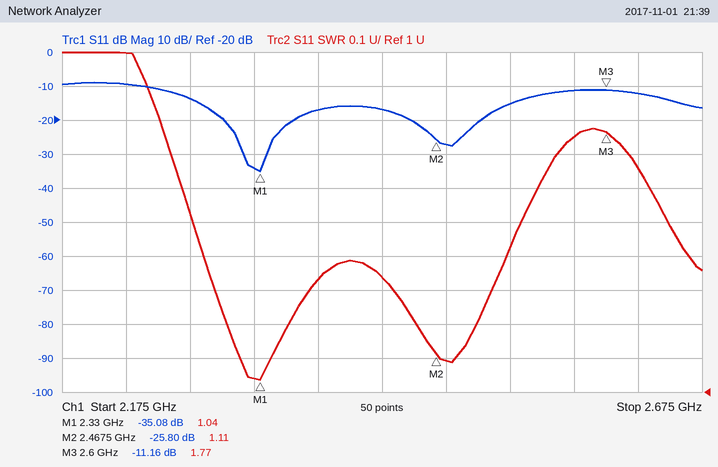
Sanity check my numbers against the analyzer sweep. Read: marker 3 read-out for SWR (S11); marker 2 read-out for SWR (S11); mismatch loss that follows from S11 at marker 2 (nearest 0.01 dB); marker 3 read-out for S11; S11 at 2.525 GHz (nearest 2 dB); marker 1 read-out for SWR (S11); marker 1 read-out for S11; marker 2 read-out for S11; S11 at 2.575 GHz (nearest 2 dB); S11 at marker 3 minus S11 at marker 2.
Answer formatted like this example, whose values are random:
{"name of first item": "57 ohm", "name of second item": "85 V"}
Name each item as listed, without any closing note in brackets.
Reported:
{"marker 3 read-out for SWR": "1.77", "marker 2 read-out for SWR": "1.11", "mismatch loss that follows from S11 at marker 2": "0.01 dB", "marker 3 read-out for S11": "-11.16 dB", "S11 at 2.525 GHz": "-16 dB", "marker 1 read-out for SWR": "1.04", "marker 1 read-out for S11": "-35.08 dB", "marker 2 read-out for S11": "-25.80 dB", "S11 at 2.575 GHz": "-12 dB", "S11 at marker 3 minus S11 at marker 2": "14.64 dB"}
